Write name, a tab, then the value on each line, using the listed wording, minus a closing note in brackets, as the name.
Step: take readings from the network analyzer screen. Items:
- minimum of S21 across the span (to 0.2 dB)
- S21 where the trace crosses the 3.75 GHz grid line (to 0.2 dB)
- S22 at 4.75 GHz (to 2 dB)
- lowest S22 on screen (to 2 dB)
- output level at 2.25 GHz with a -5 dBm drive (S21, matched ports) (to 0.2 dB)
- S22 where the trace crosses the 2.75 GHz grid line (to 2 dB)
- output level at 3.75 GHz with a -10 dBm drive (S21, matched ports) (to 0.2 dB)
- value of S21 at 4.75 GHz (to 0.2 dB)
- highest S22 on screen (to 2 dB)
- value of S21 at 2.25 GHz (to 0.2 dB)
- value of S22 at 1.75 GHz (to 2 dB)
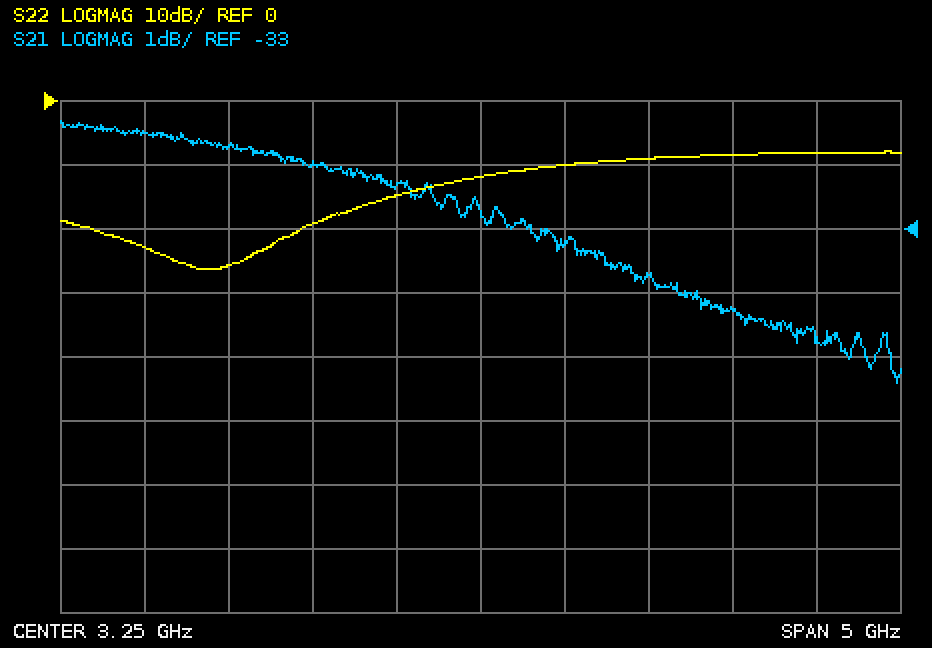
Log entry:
minimum of S21 across the span	-35.4 dB
S21 where the trace crosses the 3.75 GHz grid line	-33.2 dB
S22 at 4.75 GHz	-8 dB
lowest S22 on screen	-26 dB
output level at 2.25 GHz with a -5 dBm drive (S21, matched ports)	-37.0 dBm
S22 where the trace crosses the 2.75 GHz grid line	-14 dB
output level at 3.75 GHz with a -10 dBm drive (S21, matched ports)	-43.2 dBm
value of S21 at 4.75 GHz	-34.2 dB
highest S22 on screen	-8 dB
value of S21 at 2.25 GHz	-32.0 dB
value of S22 at 1.75 GHz	-26 dB
